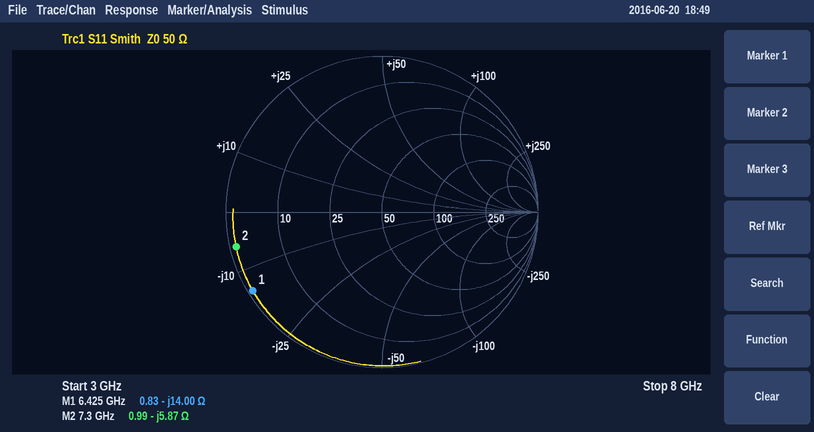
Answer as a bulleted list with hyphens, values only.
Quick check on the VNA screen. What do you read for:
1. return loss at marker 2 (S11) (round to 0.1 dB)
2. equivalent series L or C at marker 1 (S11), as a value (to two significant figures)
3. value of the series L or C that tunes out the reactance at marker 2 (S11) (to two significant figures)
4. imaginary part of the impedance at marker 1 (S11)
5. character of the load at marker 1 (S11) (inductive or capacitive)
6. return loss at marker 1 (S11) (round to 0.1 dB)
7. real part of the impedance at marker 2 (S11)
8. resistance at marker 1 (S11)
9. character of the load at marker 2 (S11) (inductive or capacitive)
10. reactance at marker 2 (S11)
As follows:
- 0.3 dB
- 1.8 pF
- 130 pH
- -14.00 Ω
- capacitive
- 0.3 dB
- 0.99 Ω
- 0.83 Ω
- capacitive
- -5.87 Ω
